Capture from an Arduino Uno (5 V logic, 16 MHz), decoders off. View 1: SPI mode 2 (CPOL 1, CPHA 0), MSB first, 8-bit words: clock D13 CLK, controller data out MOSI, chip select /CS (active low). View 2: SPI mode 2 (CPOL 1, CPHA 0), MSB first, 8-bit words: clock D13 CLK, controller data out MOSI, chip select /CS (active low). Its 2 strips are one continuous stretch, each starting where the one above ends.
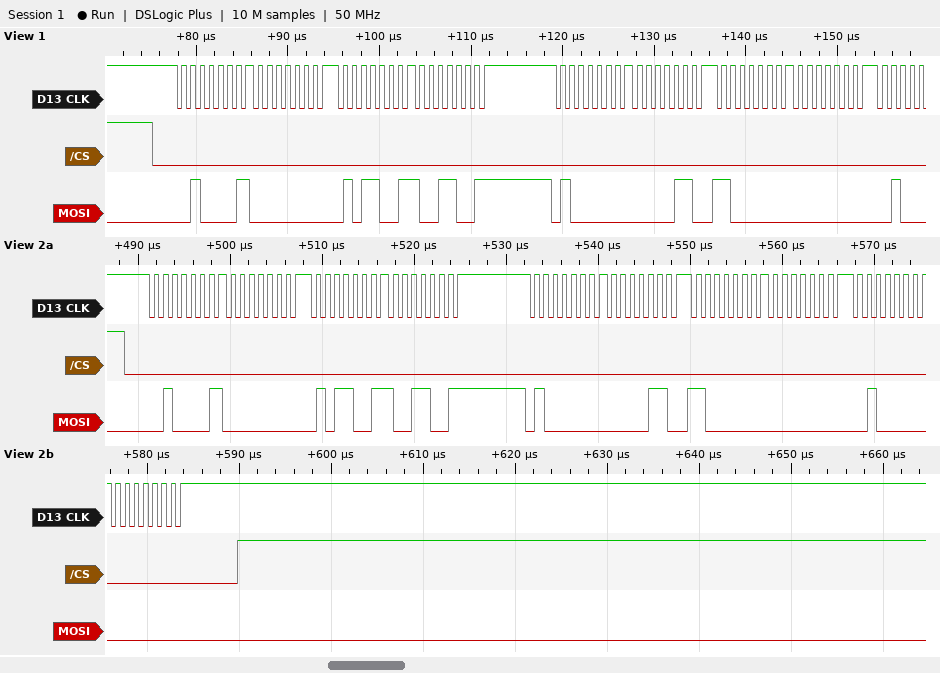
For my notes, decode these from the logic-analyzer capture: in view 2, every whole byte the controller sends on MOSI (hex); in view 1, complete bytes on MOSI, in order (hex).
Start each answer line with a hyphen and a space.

- 21 00 59 99 40 06 C0 00 20 00
- 21 00 59 99 40 06 C0 00
